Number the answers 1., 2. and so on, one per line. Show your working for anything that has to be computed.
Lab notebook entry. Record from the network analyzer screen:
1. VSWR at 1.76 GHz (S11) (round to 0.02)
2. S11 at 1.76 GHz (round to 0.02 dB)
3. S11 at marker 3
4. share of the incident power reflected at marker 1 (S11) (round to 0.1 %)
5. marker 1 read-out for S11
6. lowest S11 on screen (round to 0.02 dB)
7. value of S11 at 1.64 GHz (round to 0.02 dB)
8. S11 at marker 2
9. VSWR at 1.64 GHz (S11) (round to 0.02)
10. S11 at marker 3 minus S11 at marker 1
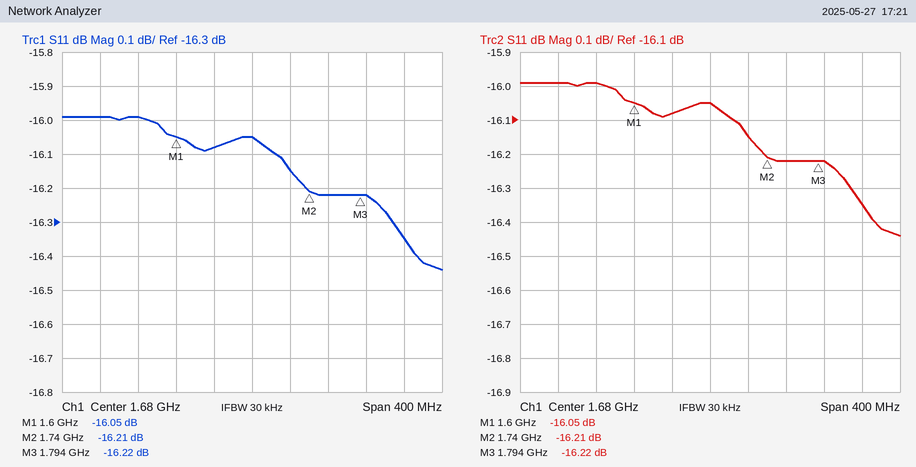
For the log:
1. |Γ| = 10^(-16.22/20) = 0.1545; VSWR = (1 + 0.1545)/(1 − 0.1545) ≈ 1.37, so 1.36 to the nearest 0.02
2. -16.22 dB
3. -16.22 dB
4. 10^(-16.05/10) ≈ 2.5 %
5. -16.05 dB
6. -16.44 dB
7. -16.08 dB
8. -16.21 dB
9. |Γ| = 10^(-16.08/20) = 0.1570; VSWR = (1 + 0.1570)/(1 − 0.1570) ≈ 1.37, so 1.38 to the nearest 0.02
10. -16.22 − (-16.05) = -0.17 dB
